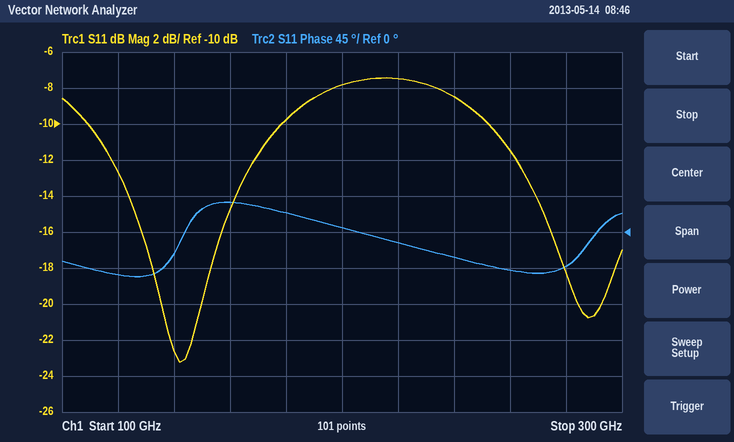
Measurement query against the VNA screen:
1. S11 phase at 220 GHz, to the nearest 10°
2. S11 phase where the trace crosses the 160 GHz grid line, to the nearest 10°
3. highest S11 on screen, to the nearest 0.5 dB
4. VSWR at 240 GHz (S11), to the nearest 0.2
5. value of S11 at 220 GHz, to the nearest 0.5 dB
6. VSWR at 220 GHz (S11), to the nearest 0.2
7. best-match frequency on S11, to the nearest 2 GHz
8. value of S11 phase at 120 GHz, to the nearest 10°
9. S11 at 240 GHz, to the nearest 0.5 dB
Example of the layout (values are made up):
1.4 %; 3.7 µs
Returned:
-10°; 40°; -7.5 dB; 2.2; -7.5 dB; 2.4; 142 GHz; -50°; -8.5 dB
